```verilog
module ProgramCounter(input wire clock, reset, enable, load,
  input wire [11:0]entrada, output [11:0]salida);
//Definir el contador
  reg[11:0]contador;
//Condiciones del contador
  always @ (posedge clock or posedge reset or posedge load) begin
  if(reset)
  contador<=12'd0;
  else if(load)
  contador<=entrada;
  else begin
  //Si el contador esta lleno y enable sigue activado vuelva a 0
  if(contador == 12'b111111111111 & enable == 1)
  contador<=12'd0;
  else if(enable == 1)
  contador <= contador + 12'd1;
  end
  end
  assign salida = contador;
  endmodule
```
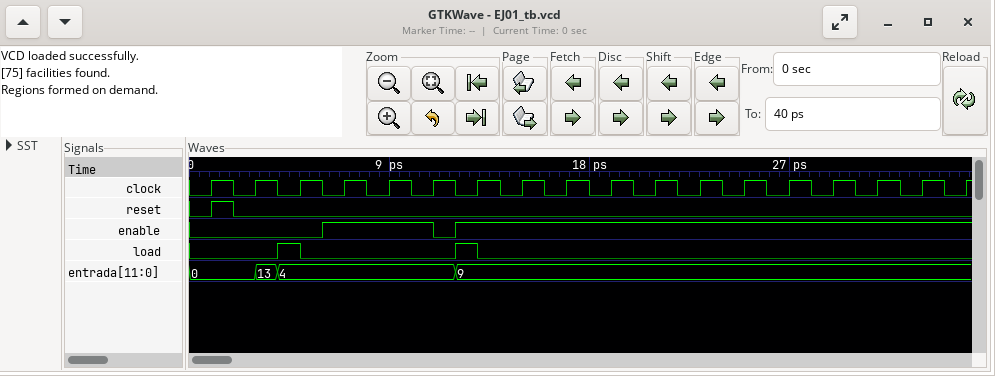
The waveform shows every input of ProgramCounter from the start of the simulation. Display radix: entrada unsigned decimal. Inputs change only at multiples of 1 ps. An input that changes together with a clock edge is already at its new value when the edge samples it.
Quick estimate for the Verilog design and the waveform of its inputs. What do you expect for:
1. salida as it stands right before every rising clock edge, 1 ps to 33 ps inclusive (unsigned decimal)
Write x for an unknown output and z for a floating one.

x, 0, 4, 4, 5, 6, 9, 10, 11, 12, 13, 14, 15, 16, 17, 18, 19
